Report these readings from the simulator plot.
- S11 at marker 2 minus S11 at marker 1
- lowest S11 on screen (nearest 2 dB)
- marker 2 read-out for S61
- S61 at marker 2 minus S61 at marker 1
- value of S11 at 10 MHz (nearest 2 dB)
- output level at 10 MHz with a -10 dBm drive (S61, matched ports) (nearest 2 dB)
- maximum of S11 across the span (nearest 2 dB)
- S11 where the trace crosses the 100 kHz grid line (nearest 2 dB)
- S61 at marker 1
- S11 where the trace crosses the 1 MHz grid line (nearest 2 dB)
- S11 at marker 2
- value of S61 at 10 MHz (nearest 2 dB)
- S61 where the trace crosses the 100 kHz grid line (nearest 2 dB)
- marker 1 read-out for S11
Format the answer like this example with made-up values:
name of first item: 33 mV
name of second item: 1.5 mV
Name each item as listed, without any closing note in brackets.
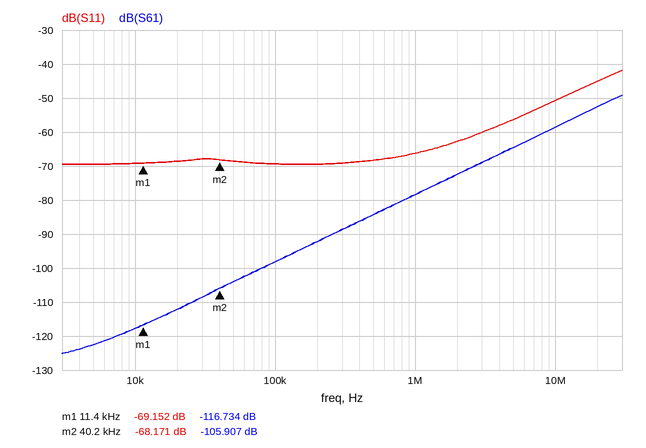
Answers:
S11 at marker 2 minus S11 at marker 1: 0.981 dB
lowest S11 on screen: -70 dB
marker 2 read-out for S61: -105.907 dB
S61 at marker 2 minus S61 at marker 1: 10.827 dB
value of S11 at 10 MHz: -50 dB
output level at 10 MHz with a -10 dBm drive (S61, matched ports): -68 dBm
maximum of S11 across the span: -42 dB
S11 where the trace crosses the 100 kHz grid line: -70 dB
S61 at marker 1: -116.734 dB
S11 where the trace crosses the 1 MHz grid line: -66 dB
S11 at marker 2: -68.171 dB
value of S61 at 10 MHz: -58 dB
S61 where the trace crosses the 100 kHz grid line: -98 dB
marker 1 read-out for S11: -69.152 dB
